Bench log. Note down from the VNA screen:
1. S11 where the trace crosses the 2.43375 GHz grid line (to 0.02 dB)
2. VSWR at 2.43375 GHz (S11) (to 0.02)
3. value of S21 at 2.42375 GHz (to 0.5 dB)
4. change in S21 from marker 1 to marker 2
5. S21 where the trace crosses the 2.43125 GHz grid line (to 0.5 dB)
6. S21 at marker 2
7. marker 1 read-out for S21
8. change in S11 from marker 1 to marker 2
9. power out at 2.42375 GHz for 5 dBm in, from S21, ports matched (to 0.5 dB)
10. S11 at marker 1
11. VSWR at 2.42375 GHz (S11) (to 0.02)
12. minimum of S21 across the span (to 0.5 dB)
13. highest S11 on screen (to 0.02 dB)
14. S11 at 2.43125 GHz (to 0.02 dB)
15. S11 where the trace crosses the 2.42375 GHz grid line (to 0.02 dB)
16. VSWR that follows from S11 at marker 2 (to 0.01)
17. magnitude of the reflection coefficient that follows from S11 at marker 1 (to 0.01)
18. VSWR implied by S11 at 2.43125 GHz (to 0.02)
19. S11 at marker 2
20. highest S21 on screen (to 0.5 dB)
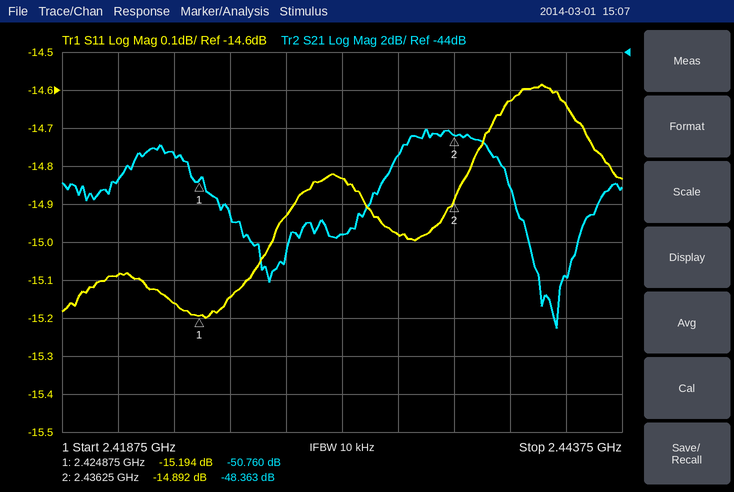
-14.98 dB
1.44
-49.5 dB
2.397 dB
-53.5 dB
-48.363 dB
-50.760 dB
0.302 dB
-44.5 dBm
-15.194 dB
1.42
-58.5 dB
-14.58 dB
-14.84 dB
-15.16 dB
1.44
0.17
1.44
-14.892 dB
-48.0 dB
